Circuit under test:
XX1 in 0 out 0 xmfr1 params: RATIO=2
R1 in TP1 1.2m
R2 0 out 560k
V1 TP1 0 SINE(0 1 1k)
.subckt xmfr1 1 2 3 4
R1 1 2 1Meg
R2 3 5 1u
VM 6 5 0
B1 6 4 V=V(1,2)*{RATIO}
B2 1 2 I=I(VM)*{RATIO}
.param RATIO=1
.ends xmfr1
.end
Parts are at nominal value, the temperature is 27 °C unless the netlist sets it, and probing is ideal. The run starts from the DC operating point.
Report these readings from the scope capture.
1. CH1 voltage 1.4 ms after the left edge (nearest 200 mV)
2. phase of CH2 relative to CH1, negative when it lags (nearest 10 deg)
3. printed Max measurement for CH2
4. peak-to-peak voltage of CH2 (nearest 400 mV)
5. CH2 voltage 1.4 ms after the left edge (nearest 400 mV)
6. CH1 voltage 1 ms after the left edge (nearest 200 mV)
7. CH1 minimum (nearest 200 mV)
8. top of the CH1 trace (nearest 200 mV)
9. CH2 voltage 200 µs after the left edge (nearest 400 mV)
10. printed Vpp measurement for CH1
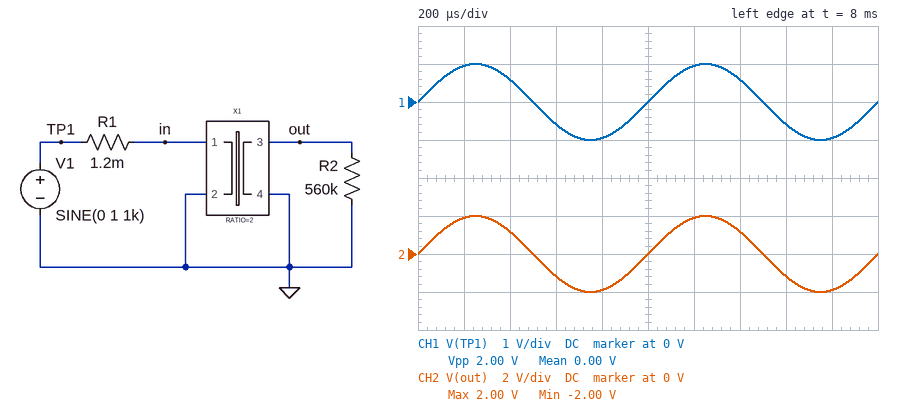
600 mV
0 deg
2.00 V
4.0 V
1.2 V
0 V
-1.0 V
1.0 V
2.0 V
2.00 V
